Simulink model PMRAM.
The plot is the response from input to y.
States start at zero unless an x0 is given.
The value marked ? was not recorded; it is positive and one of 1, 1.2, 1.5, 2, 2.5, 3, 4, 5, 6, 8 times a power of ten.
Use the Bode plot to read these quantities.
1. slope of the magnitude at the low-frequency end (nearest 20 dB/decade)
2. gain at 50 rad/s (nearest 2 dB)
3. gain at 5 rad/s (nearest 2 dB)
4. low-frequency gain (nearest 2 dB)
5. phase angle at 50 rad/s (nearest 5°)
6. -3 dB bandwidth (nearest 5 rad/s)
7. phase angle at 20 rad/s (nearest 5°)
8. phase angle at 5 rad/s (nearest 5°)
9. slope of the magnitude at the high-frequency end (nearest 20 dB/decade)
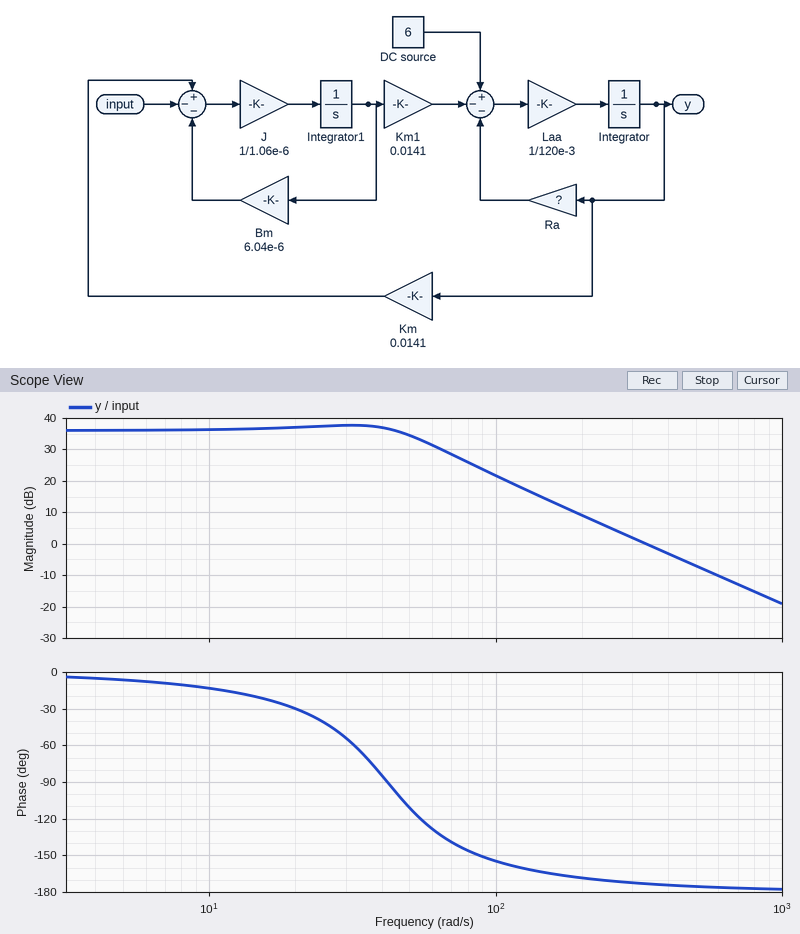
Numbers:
0 dB/decade
34 dB
36 dB
36 dB
-110°
55 rad/s
-30°
-5°
-40 dB/decade
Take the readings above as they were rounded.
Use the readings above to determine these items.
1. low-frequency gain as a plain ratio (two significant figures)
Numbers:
63
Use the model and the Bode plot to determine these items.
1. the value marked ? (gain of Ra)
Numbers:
4
